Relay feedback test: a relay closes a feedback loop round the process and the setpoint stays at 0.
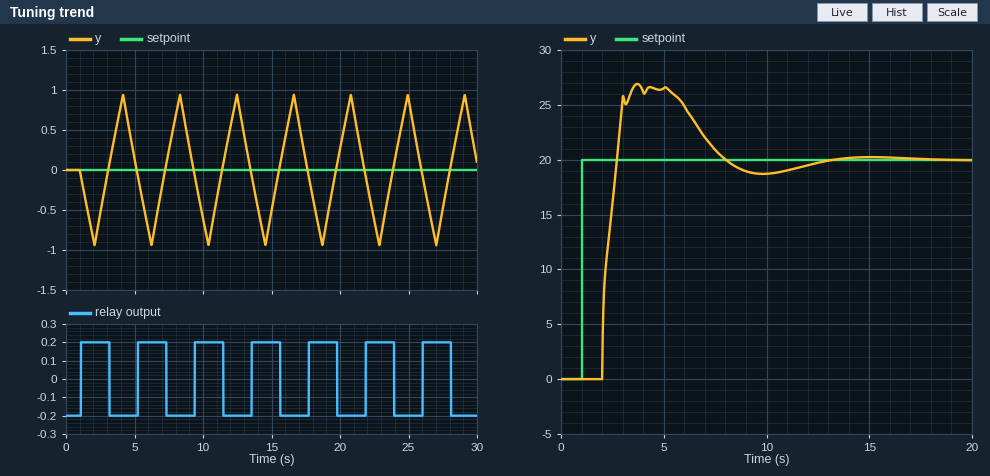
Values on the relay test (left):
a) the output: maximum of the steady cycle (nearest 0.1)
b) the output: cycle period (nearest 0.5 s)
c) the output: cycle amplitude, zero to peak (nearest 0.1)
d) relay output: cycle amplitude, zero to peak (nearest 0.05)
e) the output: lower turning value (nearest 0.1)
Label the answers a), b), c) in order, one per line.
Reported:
a) 0.9
b) 4.0 s
c) 0.9
d) 0.20
e) -0.9
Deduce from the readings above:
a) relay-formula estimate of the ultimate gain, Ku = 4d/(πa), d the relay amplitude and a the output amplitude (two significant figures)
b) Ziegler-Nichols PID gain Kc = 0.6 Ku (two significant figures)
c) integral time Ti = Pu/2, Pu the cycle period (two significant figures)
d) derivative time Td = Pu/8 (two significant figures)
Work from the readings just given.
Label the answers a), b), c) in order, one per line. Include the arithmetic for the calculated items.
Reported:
a) 4 × 0.2 / (π × 0.9) = 0.28
b) 0.6 × 0.28 = 0.17
c) 4 / 2 = 2.0 s
d) 4 / 8 = 0.50 s
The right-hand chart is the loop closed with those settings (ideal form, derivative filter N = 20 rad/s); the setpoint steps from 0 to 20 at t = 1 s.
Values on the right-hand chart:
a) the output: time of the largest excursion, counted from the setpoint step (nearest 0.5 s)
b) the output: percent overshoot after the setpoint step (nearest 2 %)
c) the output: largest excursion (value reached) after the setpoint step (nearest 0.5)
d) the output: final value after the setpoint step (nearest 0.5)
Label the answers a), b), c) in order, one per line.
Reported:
a) 2.5 s
b) 34 %
c) 27.0
d) 20.0
